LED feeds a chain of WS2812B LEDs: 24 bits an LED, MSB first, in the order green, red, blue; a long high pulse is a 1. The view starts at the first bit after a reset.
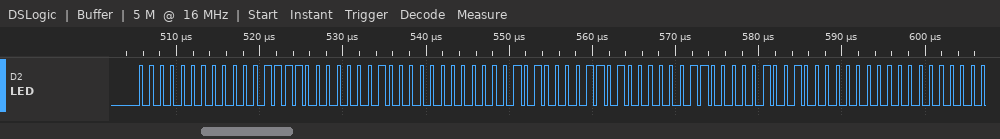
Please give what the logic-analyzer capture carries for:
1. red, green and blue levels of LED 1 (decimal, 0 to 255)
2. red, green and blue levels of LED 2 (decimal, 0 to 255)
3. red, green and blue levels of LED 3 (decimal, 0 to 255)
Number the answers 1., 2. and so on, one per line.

1. 15, 0, 1
2. 10, 0, 26
3. 9, 6, 0
